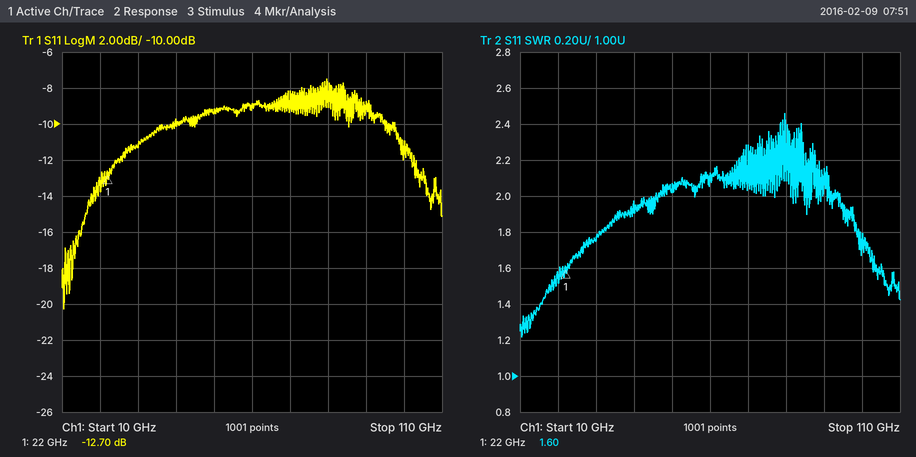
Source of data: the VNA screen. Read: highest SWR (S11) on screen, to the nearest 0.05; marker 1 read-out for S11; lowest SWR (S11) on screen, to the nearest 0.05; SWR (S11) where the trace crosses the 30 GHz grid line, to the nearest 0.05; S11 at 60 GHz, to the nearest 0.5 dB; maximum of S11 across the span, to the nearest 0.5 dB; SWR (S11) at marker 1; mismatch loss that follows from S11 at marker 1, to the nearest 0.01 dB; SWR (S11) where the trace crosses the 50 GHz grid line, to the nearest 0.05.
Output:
2.45
-12.70 dB
1.20
1.75
-9.0 dB
-7.5 dB
1.60
0.24 dB
2.05
